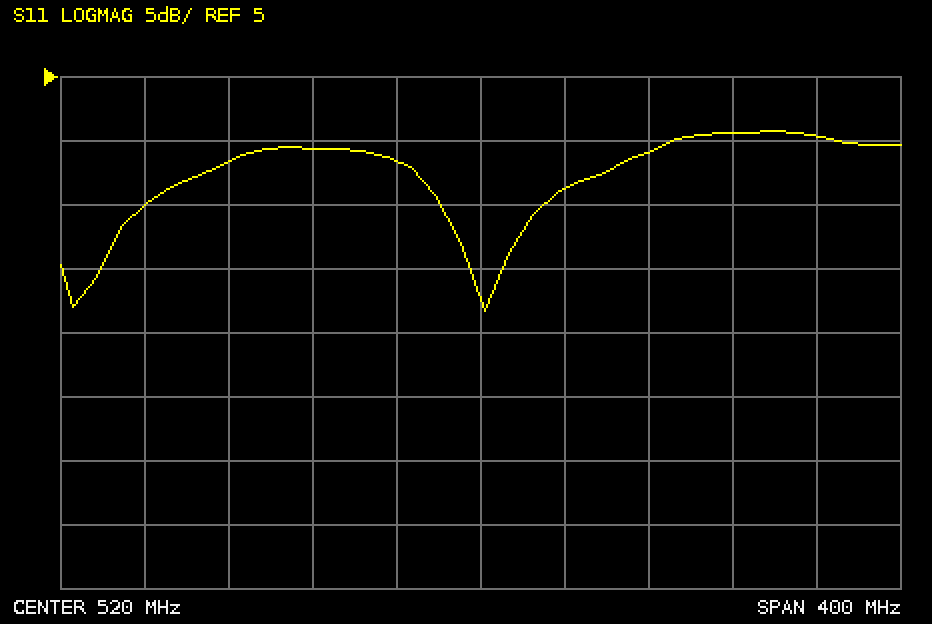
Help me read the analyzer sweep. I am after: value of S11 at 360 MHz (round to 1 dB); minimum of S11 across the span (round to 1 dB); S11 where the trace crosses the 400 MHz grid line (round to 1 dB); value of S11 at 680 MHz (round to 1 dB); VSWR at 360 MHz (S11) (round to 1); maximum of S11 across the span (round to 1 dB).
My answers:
-5 dB
-13 dB
-2 dB
0 dB
4
1 dB
